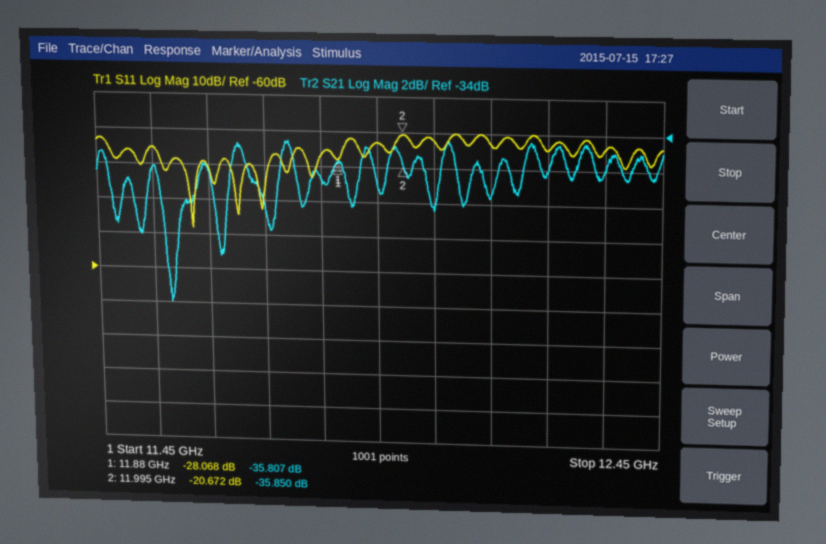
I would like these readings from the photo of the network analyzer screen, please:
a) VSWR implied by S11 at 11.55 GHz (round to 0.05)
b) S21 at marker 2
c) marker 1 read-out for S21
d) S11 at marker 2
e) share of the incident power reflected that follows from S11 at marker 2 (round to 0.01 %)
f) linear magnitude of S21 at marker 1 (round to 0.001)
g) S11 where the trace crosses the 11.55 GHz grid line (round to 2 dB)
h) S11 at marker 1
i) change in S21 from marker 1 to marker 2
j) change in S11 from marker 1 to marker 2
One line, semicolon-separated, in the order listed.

1.10; -35.850 dB; -35.807 dB; -20.672 dB; 0.86 %; 0.016; -26 dB; -28.068 dB; -0.043 dB; 7.396 dB
